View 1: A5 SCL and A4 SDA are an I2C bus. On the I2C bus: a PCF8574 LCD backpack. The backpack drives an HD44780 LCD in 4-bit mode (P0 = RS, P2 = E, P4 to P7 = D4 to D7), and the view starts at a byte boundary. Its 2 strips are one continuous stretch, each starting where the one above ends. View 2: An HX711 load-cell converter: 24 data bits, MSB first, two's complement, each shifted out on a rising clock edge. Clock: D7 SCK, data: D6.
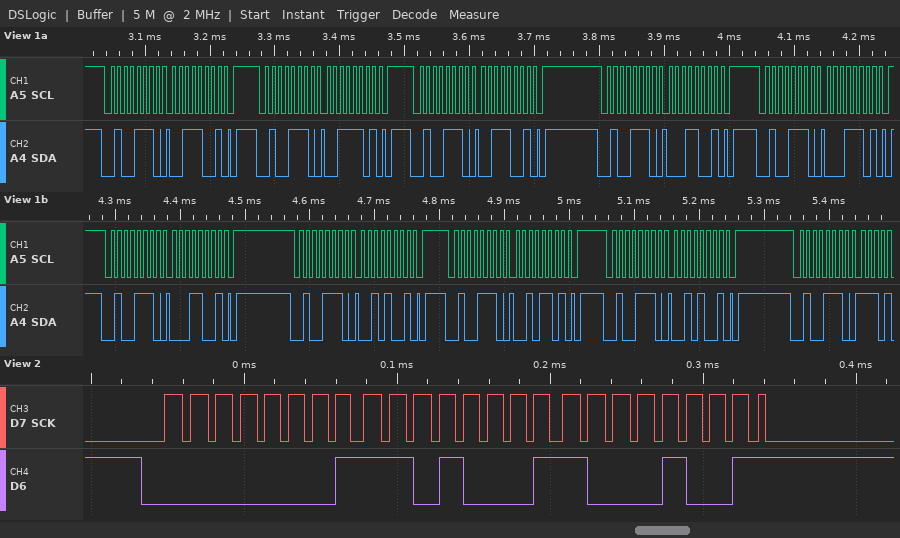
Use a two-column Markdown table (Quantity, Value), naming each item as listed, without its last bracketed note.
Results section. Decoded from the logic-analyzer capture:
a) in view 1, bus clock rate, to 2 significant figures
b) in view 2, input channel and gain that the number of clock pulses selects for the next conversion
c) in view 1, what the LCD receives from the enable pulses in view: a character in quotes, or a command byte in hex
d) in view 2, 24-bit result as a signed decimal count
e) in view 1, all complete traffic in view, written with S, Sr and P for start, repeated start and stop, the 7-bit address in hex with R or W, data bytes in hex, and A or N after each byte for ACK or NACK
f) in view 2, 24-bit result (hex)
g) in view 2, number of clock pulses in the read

| Quantity | Value |
|---|---|
| in view 1, bus clock rate, to 2 significant figures | 100 kHz |
| in view 2, input channel and gain that the number of clock pulses selects for the next conversion | channel A, gain 128 |
| in view 1, what the LCD receives from the enable pulses in view: a character in quotes, or a command byte in hex | '1' |
| in view 2, 24-bit result as a signed decimal count | 119177 |
| in view 1, all complete traffic in view, written with S, Sr and P for start, repeated start and stop, the 7-bit address in hex with R or W, data bytes in hex, and A or N after each byte for ACK or NACK | S 27W A 39 A P S 27W A 3D A P S 27W A 39 A P S 27W A 19 A P S 27W A 1D A P S 27W A 19 A P S 27W A 29 A P S 27W A 2D A P S 27W A 29 A P S 27W A |
| in view 2, 24-bit result | 0x01D189 |
| in view 2, number of clock pulses in the read | 25 |
